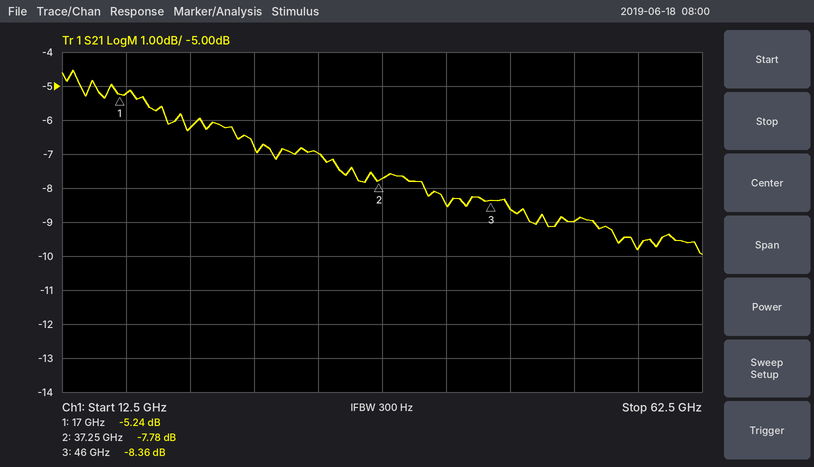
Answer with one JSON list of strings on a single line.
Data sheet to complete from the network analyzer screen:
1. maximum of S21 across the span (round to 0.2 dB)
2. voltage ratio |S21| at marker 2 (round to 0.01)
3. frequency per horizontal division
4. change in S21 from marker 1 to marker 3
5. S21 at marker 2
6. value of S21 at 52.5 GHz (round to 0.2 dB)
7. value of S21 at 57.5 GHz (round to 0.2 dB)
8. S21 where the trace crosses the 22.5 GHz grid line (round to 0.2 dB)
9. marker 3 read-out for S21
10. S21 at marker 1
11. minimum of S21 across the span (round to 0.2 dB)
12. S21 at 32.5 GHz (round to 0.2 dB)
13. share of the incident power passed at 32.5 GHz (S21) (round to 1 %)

["-4.6 dB", "0.41", "5 GHz", "-3.12 dB", "-7.78 dB", "-9.0 dB", "-9.8 dB", "-6.2 dB", "-8.36 dB", "-5.24 dB", "-10.0 dB", "-7.0 dB", "20 %"]
